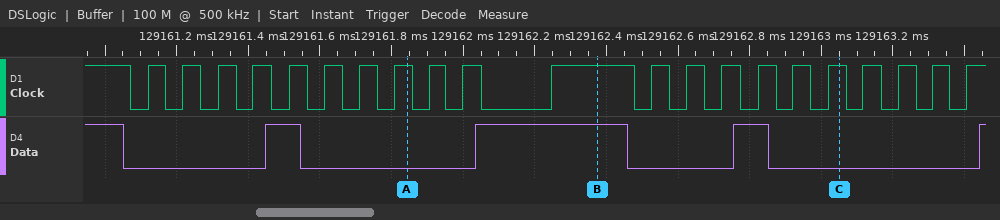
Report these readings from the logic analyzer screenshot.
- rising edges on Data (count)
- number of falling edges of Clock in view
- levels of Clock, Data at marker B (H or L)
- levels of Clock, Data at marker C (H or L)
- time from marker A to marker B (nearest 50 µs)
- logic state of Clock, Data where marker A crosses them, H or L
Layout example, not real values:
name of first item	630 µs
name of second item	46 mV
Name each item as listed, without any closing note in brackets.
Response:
rising edges on Data	4
number of falling edges of Clock in view	21
levels of Clock, Data at marker B	Clock=H, Data=H
levels of Clock, Data at marker C	Clock=H, Data=L
time from marker A to marker B	550 µs
logic state of Clock, Data where marker A crosses them, H or L	Clock=H, Data=L
